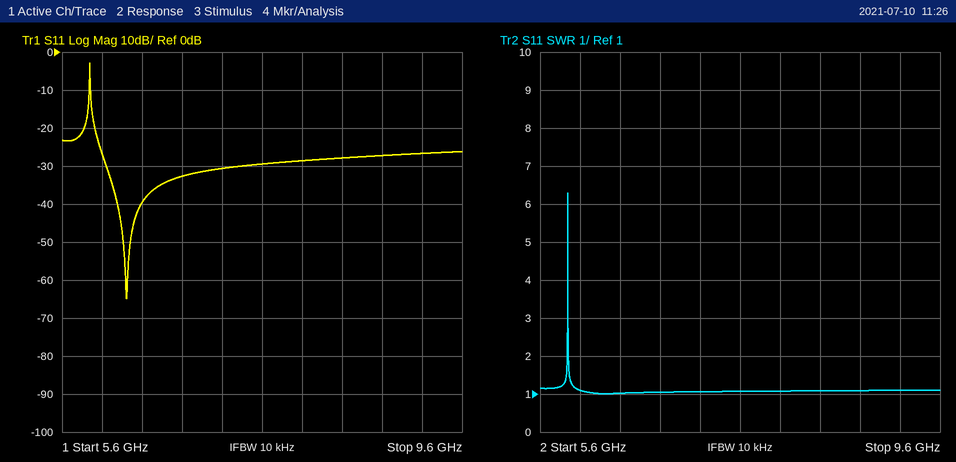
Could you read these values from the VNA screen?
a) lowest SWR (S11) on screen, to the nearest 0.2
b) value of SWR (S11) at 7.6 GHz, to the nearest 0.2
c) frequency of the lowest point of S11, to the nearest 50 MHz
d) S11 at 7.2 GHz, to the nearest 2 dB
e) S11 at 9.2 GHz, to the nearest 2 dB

1.0
1.0
6.25 GHz
-30 dB
-26 dB
